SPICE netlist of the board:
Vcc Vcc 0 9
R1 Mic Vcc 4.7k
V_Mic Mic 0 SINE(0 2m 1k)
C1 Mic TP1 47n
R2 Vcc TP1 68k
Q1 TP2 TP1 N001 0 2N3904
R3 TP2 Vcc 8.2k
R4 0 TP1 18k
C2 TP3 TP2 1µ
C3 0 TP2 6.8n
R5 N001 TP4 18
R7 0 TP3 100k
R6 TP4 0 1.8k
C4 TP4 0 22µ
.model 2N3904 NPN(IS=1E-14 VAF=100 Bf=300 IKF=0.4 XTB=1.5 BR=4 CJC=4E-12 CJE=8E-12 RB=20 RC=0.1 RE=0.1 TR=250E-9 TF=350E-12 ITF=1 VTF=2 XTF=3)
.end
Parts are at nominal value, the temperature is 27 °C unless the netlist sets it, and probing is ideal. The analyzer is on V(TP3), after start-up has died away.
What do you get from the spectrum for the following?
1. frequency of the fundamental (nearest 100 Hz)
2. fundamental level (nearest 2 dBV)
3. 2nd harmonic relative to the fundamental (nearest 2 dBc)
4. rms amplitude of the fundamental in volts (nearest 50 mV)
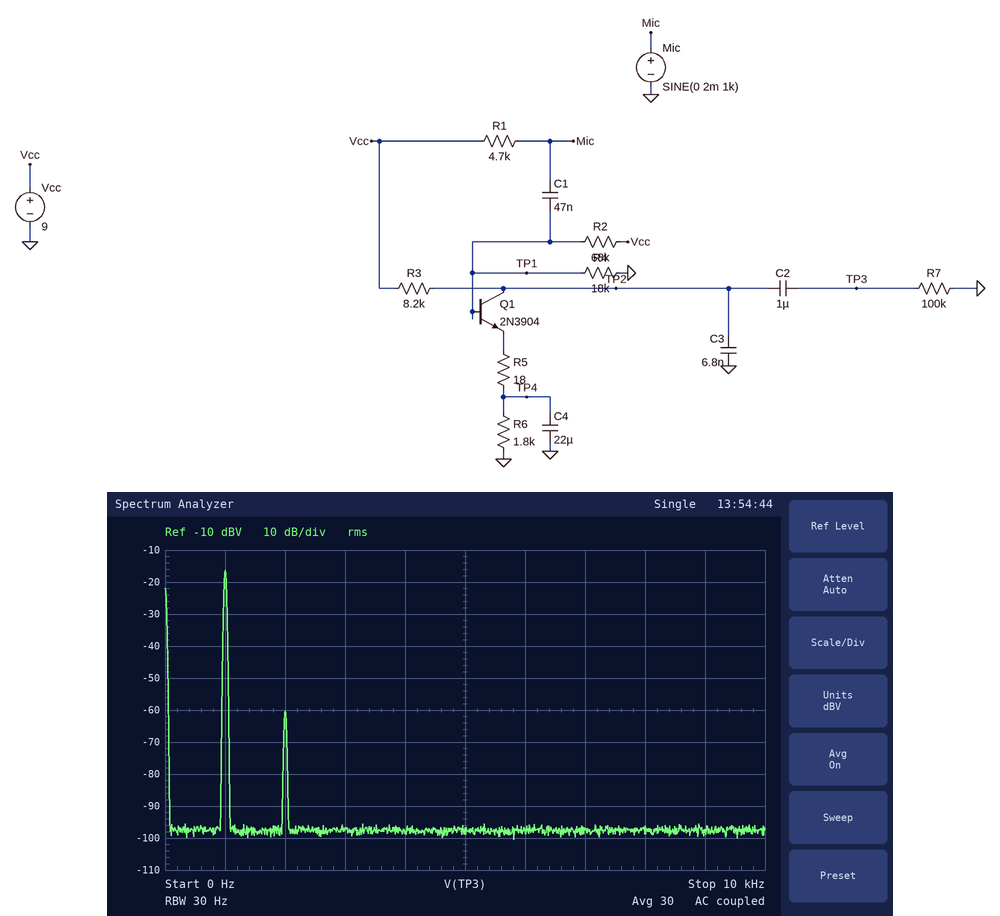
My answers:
1.0 kHz
-16 dBV
-44 dBc
150 mV
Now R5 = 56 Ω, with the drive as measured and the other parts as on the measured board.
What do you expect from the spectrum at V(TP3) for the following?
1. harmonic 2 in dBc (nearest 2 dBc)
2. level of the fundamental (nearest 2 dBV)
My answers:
-52 dBc
-20 dBV
